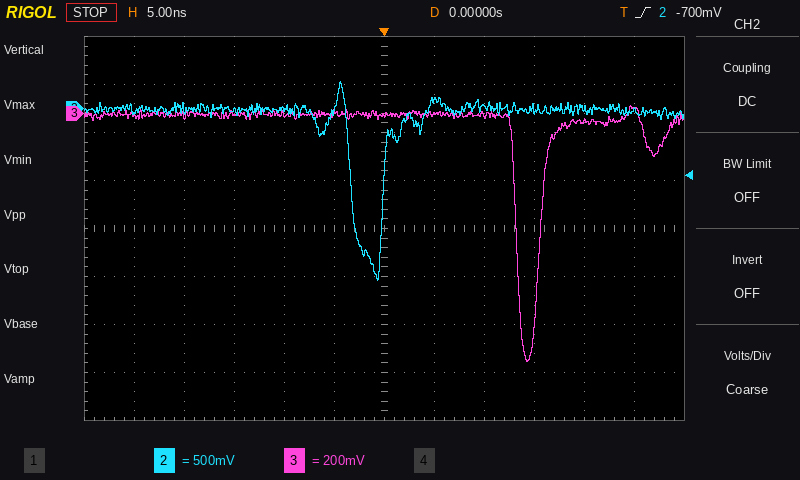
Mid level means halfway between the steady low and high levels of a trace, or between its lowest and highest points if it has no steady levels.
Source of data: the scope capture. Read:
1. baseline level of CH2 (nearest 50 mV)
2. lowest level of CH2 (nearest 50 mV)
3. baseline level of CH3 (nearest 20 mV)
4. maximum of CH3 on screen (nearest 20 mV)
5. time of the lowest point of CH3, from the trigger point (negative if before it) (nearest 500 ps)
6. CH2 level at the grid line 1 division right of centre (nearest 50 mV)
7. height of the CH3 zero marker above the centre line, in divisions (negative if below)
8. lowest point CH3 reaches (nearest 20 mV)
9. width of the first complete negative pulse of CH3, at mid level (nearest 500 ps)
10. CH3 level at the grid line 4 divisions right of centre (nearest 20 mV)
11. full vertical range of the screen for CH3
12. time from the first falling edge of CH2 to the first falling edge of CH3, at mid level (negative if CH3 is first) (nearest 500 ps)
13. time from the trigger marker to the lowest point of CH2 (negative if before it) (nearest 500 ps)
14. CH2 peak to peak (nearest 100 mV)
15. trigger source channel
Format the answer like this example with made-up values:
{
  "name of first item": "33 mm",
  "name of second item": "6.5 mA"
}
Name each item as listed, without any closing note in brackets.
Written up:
{
  "baseline level of CH2": "0 mV",
  "lowest level of CH2": "-1.80 V",
  "baseline level of CH3": "0 mV",
  "maximum of CH3 on screen": "40 mV",
  "time of the lowest point of CH3, from the trigger point (negative if before it)": "+14.5 ns",
  "CH2 level at the grid line 1 division right of centre": "100 mV",
  "height of the CH3 zero marker above the centre line, in divisions": "+2.4 div",
  "lowest point CH3 reaches": "-1.04 V",
  "width of the first complete negative pulse of CH3, at mid level": "2.5 ns",
  "CH3 level at the grid line 4 divisions right of centre": "-40 mV",
  "full vertical range of the screen for CH3": "1.6 V",
  "time from the first falling edge of CH2 to the first falling edge of CH3, at mid level (negative if CH3 is first)": "+16.5 ns",
  "time from the trigger marker to the lowest point of CH2 (negative if before it)": "-500 ps",
  "CH2 peak to peak": "2.10 V",
  "trigger source channel": "CH2"
}
